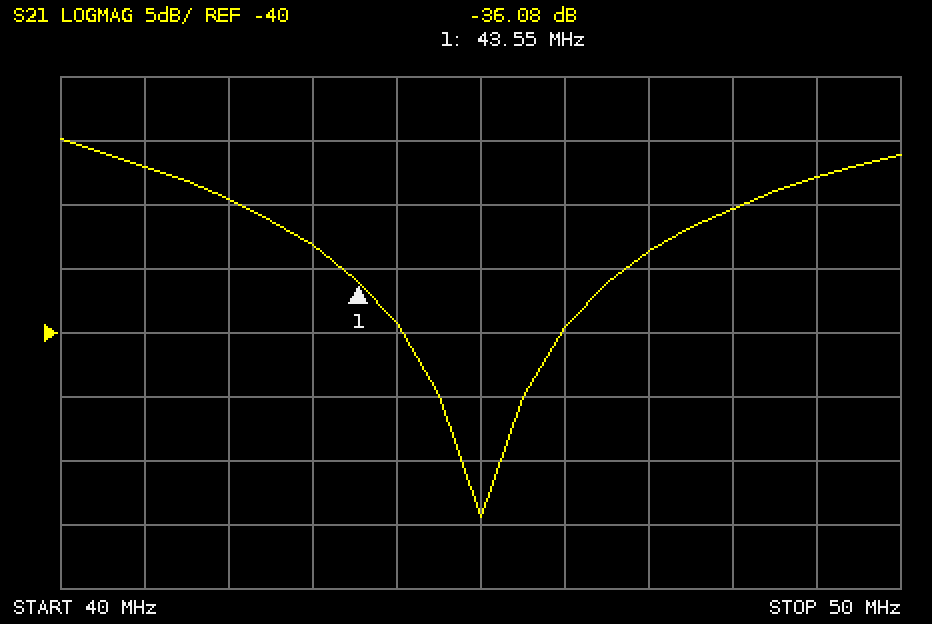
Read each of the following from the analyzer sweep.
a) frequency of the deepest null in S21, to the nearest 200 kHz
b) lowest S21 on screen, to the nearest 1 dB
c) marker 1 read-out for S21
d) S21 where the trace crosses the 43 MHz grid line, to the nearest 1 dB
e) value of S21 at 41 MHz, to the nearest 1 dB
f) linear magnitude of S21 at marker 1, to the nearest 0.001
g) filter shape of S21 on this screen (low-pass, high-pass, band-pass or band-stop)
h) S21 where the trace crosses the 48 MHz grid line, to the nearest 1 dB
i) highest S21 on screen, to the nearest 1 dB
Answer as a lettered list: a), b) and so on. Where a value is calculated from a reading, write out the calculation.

a) 45.0 MHz
b) -54 dB
c) -36.08 dB
d) -33 dB
e) -27 dB
f) 10^(-36.08/20) ≈ 0.016
g) band-stop
h) -30 dB
i) -25 dB
